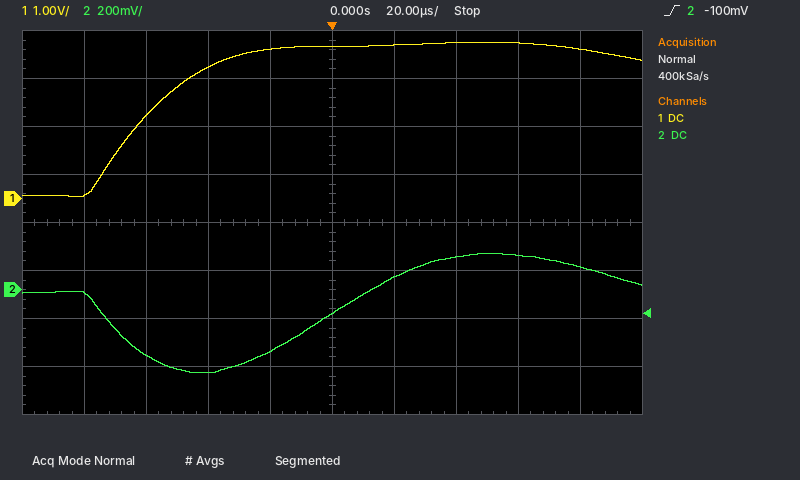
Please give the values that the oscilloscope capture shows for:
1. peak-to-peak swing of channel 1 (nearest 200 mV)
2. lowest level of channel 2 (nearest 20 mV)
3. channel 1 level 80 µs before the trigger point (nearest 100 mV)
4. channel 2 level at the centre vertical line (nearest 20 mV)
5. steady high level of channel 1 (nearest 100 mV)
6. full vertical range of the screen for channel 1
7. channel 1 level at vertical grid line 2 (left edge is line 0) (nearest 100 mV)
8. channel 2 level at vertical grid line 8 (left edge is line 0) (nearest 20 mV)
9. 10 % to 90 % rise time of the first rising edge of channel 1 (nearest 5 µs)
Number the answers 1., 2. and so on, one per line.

1. 3.2 V
2. -340 mV
3. 100 mV
4. -100 mV
5. 3.2 V
6. 8 V
7. 1.7 V
8. 140 mV
9. 40 µs
